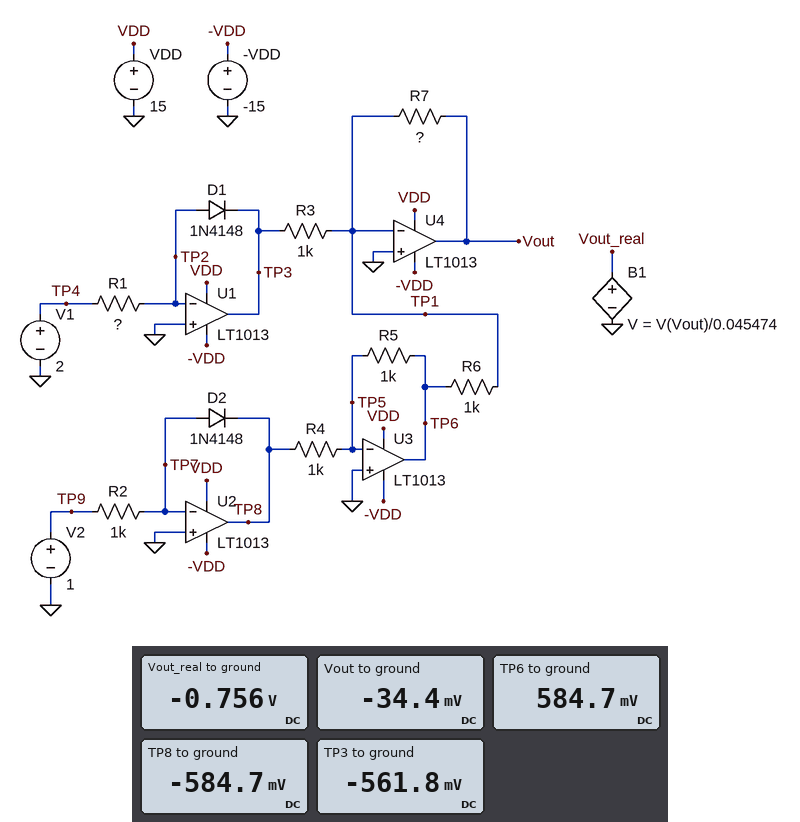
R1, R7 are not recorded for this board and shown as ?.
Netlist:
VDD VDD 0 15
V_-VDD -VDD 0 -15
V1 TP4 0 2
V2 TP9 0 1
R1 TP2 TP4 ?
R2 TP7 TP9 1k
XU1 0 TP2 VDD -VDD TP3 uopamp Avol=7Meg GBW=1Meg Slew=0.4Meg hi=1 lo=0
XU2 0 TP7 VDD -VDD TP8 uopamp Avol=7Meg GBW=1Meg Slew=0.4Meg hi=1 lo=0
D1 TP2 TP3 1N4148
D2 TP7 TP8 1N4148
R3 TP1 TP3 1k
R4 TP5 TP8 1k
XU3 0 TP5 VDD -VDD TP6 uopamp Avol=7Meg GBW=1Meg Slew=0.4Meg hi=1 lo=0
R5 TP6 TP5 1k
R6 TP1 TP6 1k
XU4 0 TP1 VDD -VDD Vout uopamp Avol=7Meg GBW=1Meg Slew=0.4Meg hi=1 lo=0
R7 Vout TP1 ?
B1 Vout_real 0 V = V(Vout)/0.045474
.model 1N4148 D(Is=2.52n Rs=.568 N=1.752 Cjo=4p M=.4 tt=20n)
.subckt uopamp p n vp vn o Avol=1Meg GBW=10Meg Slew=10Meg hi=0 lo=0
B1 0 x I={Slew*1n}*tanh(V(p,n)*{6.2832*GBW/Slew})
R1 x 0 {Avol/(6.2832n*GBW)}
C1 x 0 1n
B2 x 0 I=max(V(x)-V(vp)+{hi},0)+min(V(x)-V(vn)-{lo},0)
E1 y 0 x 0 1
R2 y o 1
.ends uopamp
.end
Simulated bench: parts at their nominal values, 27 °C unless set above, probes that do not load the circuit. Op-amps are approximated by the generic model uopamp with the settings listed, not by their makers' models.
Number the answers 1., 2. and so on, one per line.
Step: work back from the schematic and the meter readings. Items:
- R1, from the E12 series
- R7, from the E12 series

1. 3.3 kΩ
2. 1.5 kΩ
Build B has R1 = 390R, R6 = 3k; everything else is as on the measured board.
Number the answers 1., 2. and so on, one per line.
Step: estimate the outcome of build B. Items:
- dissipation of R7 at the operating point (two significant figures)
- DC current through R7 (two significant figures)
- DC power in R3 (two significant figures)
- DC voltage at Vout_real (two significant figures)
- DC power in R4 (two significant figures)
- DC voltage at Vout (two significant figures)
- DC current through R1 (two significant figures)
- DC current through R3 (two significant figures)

1. 330 µW
2. 470 µA
3. 440 µW
4. 15 V
5. 340 µW
6. 700 mV
7. 5.1 mA
8. 660 µA
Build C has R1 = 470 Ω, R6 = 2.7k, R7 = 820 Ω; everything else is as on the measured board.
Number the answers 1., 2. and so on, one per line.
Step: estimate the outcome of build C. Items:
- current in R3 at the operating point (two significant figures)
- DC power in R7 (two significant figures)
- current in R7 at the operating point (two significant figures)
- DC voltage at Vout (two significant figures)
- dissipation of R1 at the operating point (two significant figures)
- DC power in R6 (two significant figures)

1. 650 µA
2. 160 µW
3. 440 µA
4. 360 mV
5. 8.5 mW
6. 130 µW
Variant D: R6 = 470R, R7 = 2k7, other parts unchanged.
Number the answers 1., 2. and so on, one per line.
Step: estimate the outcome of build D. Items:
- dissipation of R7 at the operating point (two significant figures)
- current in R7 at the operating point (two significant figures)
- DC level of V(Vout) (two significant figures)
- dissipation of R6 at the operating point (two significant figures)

1. 1.3 mW
2. 680 µA
3. -1.8 V
4. 730 µW
